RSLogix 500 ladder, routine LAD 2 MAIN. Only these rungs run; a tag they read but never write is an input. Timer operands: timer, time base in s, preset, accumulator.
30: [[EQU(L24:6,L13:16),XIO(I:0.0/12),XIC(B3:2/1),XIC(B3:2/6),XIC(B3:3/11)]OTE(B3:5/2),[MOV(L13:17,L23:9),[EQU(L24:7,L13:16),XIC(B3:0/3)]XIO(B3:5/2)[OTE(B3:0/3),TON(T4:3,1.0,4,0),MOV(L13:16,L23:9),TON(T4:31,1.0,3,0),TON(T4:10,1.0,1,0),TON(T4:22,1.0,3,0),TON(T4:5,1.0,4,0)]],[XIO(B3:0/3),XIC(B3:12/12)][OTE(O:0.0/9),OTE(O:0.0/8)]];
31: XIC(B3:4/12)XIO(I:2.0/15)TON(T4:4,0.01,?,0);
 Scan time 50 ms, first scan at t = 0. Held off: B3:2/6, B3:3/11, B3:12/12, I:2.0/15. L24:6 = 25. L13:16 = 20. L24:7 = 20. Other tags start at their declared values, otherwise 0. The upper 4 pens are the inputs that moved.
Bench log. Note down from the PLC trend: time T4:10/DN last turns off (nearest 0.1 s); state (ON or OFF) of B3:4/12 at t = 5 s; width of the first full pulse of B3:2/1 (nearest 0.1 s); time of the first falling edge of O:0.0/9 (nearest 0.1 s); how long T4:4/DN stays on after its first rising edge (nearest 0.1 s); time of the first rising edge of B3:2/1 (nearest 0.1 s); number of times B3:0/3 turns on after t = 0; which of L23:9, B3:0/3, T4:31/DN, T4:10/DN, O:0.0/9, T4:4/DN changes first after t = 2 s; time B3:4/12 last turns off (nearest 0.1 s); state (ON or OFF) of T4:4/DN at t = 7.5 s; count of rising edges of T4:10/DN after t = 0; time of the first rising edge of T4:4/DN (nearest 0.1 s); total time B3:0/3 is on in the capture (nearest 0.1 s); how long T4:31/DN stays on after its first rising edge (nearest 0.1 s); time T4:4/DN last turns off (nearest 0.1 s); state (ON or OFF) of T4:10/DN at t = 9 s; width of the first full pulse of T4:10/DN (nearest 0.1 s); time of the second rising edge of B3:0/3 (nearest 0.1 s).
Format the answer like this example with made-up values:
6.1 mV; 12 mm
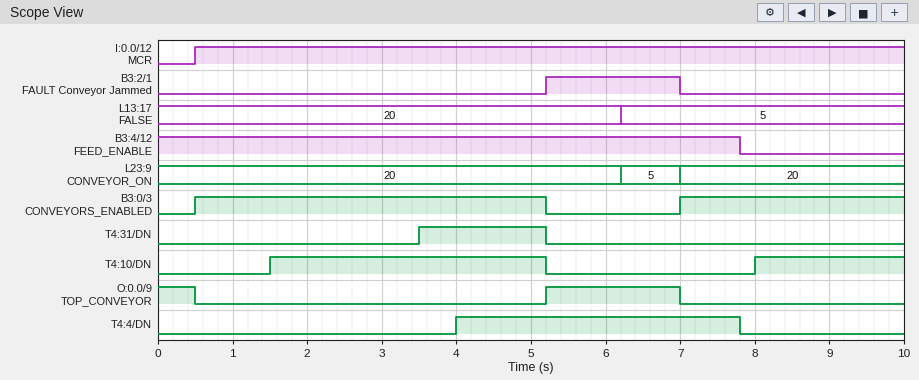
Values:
5.2 s; ON; 1.8 s; 0.5 s; 3.8 s; 5.2 s; 2; T4:31/DN; 7.8 s; ON; 2; 4.0 s; 7.7 s; 1.7 s; 7.8 s; ON; 3.7 s; 7.0 s
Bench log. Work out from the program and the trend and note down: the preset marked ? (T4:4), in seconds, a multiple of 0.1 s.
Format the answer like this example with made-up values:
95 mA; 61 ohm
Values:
4.0 s
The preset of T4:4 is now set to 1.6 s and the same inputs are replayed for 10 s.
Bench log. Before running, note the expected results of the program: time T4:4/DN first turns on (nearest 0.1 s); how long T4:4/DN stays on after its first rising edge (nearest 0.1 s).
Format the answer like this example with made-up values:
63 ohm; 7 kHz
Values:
1.6 s; 6.2 s
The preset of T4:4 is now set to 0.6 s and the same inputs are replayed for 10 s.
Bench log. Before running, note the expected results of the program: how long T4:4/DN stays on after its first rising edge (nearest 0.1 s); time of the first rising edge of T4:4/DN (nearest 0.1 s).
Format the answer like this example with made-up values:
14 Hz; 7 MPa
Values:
7.2 s; 0.6 s
